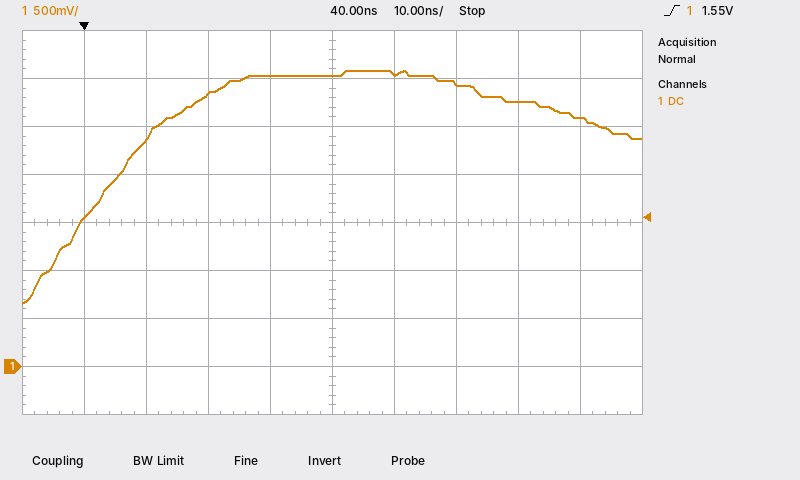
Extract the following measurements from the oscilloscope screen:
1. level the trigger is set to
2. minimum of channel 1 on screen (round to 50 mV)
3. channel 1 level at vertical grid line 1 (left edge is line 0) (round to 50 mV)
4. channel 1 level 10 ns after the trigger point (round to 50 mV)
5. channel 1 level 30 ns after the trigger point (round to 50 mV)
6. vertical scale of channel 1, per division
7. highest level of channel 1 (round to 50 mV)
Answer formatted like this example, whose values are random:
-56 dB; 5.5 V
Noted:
1.55 V; 650 mV; 1.55 V; 2.35 V; 3.05 V; 500 mV; 3.10 V
